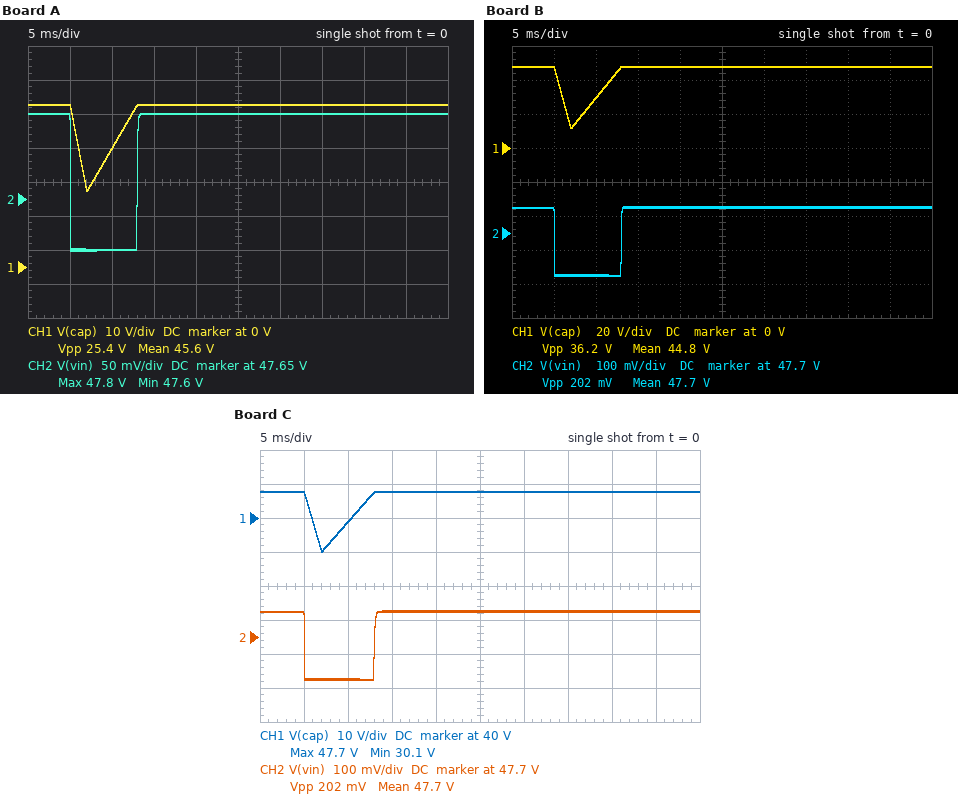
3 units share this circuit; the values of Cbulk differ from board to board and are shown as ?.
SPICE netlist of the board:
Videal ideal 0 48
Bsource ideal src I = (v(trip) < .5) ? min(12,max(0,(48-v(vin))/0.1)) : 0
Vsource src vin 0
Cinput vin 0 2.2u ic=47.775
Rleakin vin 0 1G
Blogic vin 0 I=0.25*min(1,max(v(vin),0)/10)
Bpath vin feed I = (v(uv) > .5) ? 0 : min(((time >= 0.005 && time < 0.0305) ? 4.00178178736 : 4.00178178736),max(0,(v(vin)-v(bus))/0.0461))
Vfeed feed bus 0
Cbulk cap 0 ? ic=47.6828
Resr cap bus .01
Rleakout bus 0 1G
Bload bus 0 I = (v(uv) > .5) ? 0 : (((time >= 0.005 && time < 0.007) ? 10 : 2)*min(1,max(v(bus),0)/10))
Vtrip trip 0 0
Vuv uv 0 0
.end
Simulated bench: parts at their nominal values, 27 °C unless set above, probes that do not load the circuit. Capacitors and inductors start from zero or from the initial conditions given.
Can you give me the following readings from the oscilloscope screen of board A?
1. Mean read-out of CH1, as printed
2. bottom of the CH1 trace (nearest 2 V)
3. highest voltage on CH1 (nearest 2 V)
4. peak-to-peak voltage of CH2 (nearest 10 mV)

45.6 V
22 V
48 V
200 mV
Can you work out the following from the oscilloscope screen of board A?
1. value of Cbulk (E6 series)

470 µF
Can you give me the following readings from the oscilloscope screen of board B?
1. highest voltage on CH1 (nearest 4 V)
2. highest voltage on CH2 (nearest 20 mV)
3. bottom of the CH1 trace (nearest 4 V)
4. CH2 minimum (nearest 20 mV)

48 V
47.78 V
12 V
47.58 V
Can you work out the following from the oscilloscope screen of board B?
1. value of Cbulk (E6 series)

330 µF
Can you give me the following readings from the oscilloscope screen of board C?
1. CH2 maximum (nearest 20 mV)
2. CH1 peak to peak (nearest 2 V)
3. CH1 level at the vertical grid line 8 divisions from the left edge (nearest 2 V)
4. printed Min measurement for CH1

47.78 V
18 V
48 V
30.1 V
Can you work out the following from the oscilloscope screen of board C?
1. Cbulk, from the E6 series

680 µF
